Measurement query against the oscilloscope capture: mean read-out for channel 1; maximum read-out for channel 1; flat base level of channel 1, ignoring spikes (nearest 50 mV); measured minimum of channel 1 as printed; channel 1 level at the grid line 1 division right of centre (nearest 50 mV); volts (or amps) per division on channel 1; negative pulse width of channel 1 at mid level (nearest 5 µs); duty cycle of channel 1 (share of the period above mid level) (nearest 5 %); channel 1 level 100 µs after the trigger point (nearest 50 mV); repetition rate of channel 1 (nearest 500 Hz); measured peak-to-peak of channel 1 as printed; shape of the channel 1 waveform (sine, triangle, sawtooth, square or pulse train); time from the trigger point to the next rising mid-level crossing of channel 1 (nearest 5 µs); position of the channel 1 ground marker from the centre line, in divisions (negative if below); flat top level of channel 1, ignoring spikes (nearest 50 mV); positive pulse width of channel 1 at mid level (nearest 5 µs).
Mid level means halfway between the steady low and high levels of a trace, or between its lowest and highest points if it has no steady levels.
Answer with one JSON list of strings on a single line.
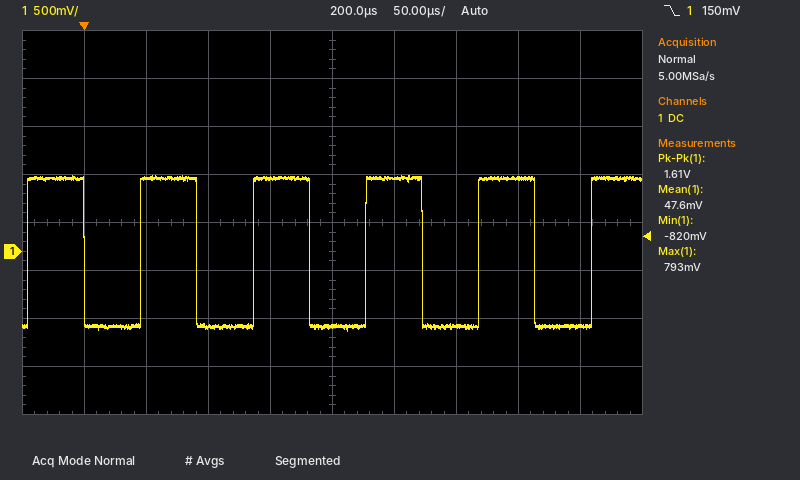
["47.6 mV", "793 mV", "-800 mV", "-820 mV", "750 mV", "500 mV", "45 µs", "50 %", "-800 mV", "11.0 kHz", "1.61 V", "square", "45 µs", "-0.6 div", "750 mV", "45 µs"]
